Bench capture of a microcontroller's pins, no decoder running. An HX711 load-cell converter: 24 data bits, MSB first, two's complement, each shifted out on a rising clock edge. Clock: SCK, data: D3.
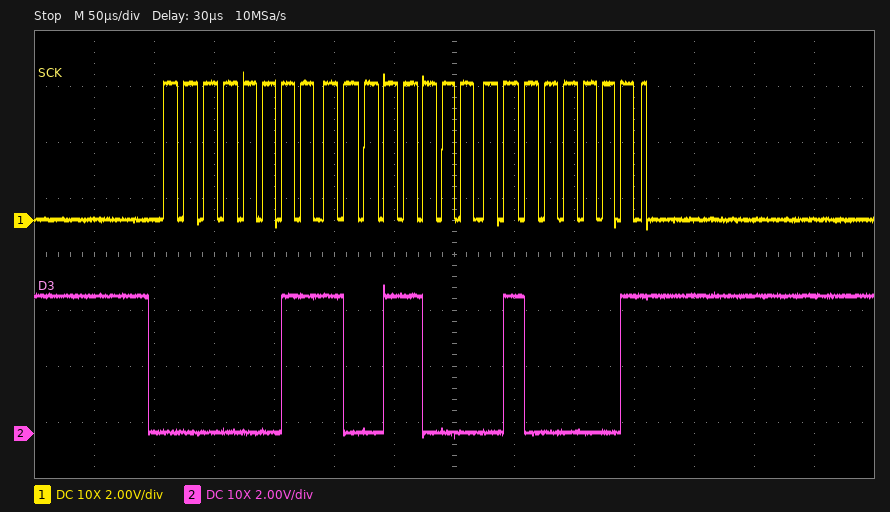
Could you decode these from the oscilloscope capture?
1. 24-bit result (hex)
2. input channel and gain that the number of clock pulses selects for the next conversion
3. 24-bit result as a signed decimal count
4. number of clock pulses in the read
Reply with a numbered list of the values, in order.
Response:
1. 0x039841
2. channel A, gain 128
3. 235585
4. 25
